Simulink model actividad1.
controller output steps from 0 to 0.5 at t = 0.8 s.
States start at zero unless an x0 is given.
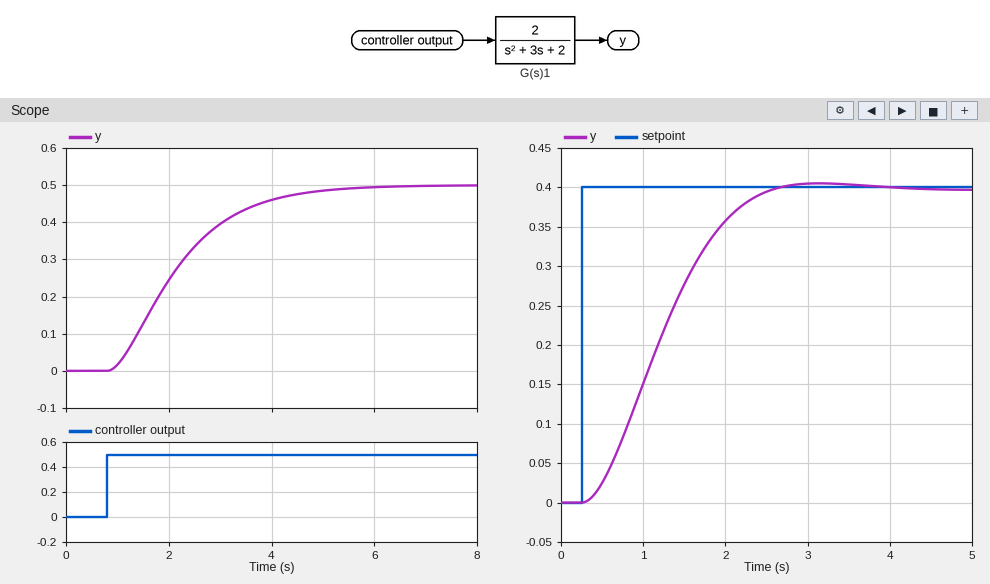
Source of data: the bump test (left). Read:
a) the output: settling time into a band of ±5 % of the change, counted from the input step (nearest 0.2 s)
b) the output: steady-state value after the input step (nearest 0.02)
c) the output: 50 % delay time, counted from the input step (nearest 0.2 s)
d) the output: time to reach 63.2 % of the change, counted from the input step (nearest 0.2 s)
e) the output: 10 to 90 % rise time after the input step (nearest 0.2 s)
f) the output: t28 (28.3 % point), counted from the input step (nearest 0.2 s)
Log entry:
3.6 s
0.50
1.2 s
1.6 s
2.6 s
0.8 s
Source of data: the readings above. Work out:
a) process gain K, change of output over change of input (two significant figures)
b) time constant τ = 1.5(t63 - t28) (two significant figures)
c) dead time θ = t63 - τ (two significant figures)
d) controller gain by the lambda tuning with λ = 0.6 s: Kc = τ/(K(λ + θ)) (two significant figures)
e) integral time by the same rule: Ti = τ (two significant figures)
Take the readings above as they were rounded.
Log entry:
1.0
1.2 s
0.40 s
1.2
1.2 s
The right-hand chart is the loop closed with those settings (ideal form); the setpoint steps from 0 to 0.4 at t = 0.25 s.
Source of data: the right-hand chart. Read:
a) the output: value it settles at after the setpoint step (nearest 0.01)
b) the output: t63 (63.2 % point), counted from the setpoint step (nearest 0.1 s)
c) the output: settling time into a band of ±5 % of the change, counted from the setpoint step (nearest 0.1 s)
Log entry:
0.40
1.1 s
2.0 s
